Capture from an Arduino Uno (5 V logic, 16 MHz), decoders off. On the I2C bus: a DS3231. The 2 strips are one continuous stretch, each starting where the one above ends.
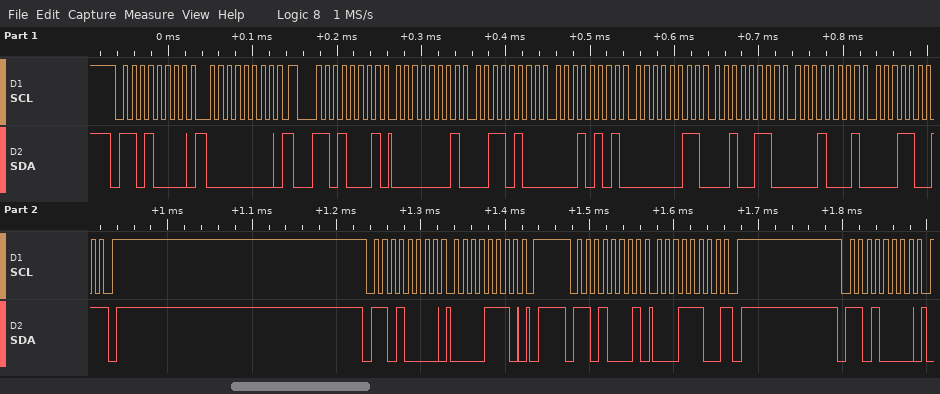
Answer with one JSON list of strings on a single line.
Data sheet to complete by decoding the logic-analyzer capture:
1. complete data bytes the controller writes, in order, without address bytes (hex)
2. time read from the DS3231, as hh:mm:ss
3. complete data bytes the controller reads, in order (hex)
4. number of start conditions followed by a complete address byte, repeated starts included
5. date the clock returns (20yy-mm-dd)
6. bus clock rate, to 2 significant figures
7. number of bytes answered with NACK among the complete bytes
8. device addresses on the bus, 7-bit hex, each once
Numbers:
["00 0E", "15:34:01", "01 34 15 03 26 11 19 1C", "5", "2019-11-26", "100 kHz", "2", "0x68"]
